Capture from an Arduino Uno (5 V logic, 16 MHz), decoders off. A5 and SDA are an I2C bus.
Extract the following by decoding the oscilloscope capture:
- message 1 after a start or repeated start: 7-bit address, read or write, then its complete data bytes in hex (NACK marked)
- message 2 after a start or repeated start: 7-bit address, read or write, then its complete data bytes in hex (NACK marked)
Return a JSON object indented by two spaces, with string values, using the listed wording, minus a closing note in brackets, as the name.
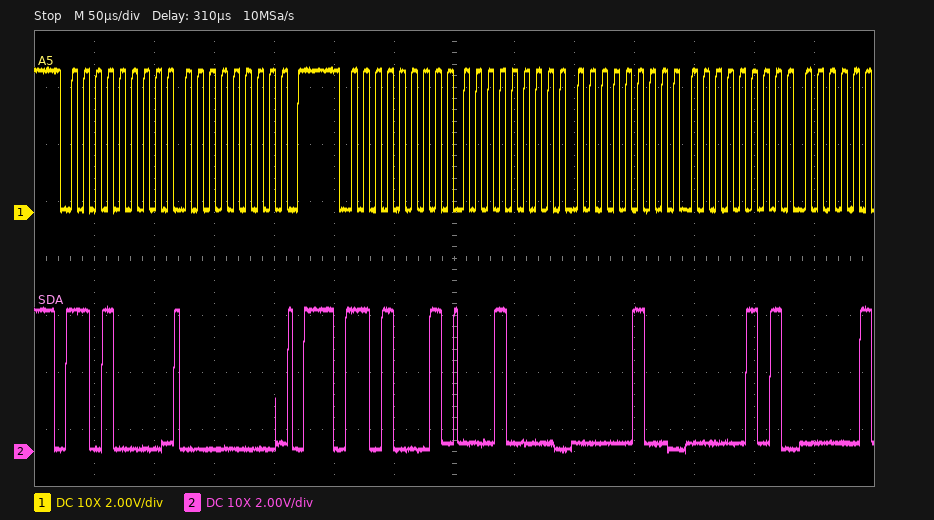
{
  "message 1 after a start or repeated start: 7-bit address, read or write, then its complete data bytes in hex": "0x68 write: 00",
  "message 2 after a start or repeated start: 7-bit address, read or write, then its complete data bytes in hex": "0x68 read: 10 04 05"
}
